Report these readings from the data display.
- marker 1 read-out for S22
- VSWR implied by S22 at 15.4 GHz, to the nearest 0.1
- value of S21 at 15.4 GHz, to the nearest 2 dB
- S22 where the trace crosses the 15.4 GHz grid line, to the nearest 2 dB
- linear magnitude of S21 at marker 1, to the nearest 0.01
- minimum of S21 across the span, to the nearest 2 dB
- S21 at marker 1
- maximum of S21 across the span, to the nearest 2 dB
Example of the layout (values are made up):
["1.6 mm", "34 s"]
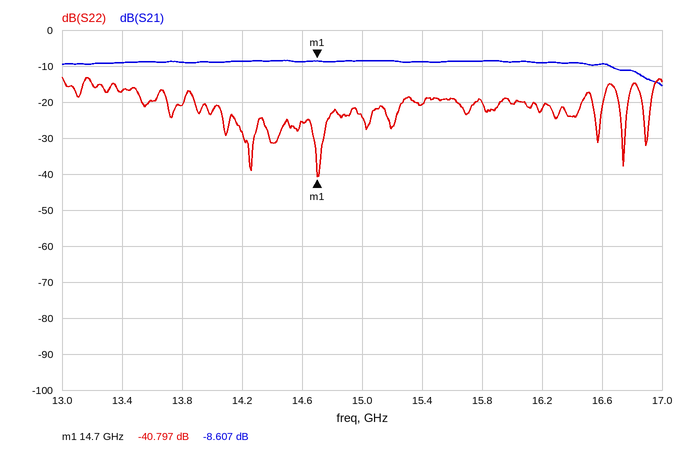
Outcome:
["-40.797 dB", "1.2", "-8 dB", "-20 dB", "0.37", "-16 dB", "-8.607 dB", "-8 dB"]
